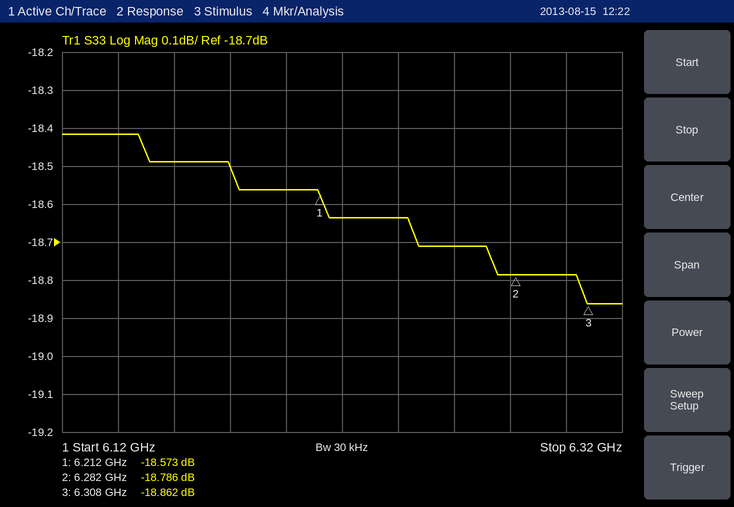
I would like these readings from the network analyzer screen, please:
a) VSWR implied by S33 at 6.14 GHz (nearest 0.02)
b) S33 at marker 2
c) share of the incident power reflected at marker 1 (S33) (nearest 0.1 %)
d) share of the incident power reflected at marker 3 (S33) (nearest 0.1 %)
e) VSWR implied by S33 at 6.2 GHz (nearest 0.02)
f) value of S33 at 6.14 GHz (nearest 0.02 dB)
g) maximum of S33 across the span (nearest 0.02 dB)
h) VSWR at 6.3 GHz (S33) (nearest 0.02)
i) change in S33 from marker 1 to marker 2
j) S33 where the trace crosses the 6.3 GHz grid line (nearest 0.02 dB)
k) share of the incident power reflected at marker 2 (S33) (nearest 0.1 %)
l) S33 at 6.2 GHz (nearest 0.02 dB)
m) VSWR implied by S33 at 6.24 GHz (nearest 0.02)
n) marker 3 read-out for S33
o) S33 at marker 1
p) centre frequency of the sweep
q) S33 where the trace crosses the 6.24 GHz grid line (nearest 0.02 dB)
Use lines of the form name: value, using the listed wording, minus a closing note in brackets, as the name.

VSWR implied by S33 at 6.14 GHz: 1.28
S33 at marker 2: -18.786 dB
share of the incident power reflected at marker 1 (S33): 1.4 %
share of the incident power reflected at marker 3 (S33): 1.3 %
VSWR implied by S33 at 6.2 GHz: 1.26
value of S33 at 6.14 GHz: -18.42 dB
maximum of S33 across the span: -18.42 dB
VSWR at 6.3 GHz (S33): 1.26
change in S33 from marker 1 to marker 2: -0.213 dB
S33 where the trace crosses the 6.3 GHz grid line: -18.78 dB
share of the incident power reflected at marker 2 (S33): 1.3 %
S33 at 6.2 GHz: -18.56 dB
VSWR implied by S33 at 6.24 GHz: 1.26
marker 3 read-out for S33: -18.862 dB
S33 at marker 1: -18.573 dB
centre frequency of the sweep: 6.22 GHz
S33 where the trace crosses the 6.24 GHz grid line: -18.64 dB
